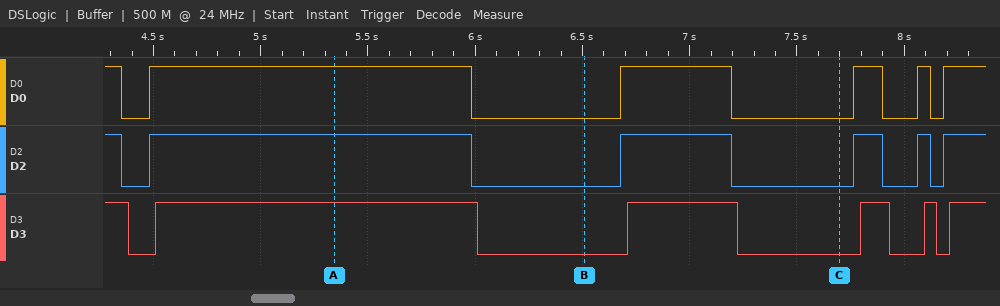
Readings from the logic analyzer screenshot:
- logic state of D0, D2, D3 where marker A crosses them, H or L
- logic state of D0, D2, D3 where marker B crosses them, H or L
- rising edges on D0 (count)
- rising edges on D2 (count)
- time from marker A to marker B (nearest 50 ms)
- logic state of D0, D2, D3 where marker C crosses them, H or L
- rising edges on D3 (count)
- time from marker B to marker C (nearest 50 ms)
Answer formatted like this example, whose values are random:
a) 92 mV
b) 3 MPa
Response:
a) D0=H, D2=H, D3=H
b) D0=L, D2=L, D3=L
c) 5
d) 5
e) 1150 ms
f) D0=L, D2=L, D3=L
g) 5
h) 1200 ms
